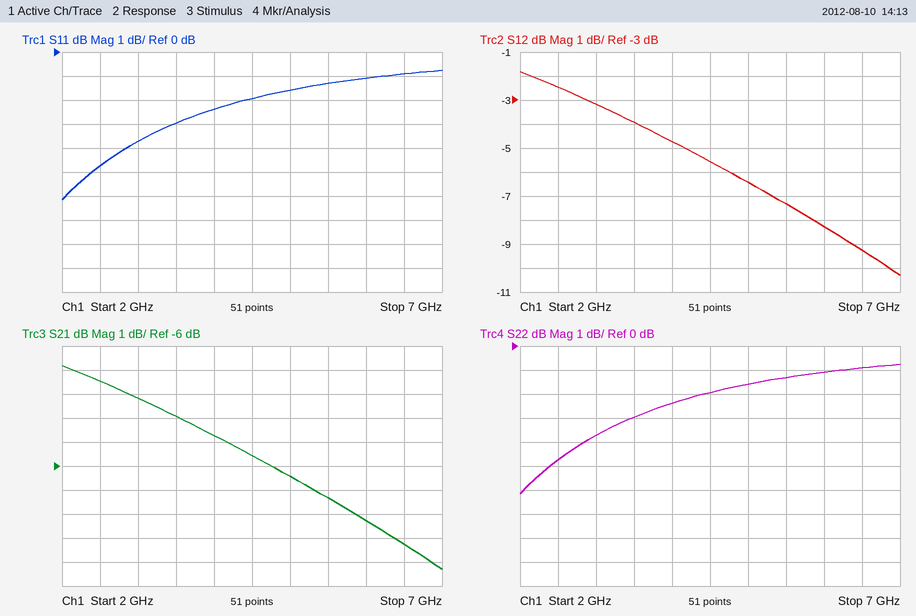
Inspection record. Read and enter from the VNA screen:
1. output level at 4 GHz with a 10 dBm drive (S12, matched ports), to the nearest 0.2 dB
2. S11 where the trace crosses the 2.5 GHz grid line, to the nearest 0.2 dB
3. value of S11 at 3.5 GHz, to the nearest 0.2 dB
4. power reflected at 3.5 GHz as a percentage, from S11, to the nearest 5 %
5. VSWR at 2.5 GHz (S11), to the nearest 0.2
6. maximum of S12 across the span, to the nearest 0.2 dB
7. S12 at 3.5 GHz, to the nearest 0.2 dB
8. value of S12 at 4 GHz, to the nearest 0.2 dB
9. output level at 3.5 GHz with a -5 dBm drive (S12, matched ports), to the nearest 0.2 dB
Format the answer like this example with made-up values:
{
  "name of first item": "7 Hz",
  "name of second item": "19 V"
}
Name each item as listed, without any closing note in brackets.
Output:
{
  "output level at 4 GHz with a 10 dBm drive (S12, matched ports), to the nearest 0.2 dB": "5.2 dBm",
  "S11 where the trace crosses the 2.5 GHz grid line, to the nearest 0.2 dB": "-4.8 dB",
  "value of S11 at 3.5 GHz, to the nearest 0.2 dB": "-3.0 dB",
  "power reflected at 3.5 GHz as a percentage, from S11, to the nearest 5 %": "50 %",
  "VSWR at 2.5 GHz (S11), to the nearest 0.2": "3.8",
  "maximum of S12 across the span, to the nearest 0.2 dB": "-1.8 dB",
  "S12 at 3.5 GHz, to the nearest 0.2 dB": "-4.0 dB",
  "value of S12 at 4 GHz, to the nearest 0.2 dB": "-4.8 dB",
  "output level at 3.5 GHz with a -5 dBm drive (S12, matched ports), to the nearest 0.2 dB": "-9.0 dBm"
}
